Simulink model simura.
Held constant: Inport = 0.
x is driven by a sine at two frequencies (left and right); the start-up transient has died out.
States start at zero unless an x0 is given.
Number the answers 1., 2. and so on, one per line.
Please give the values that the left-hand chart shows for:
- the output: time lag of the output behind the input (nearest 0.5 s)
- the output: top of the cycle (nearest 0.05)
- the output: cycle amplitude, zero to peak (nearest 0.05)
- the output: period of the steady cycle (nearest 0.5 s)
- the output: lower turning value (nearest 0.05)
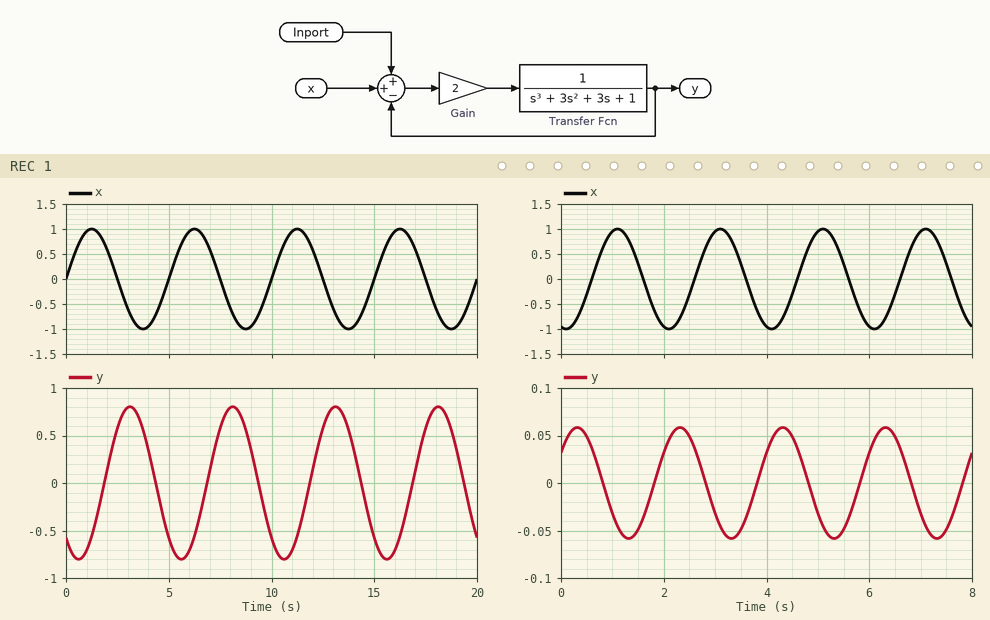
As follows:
1. 2.0 s
2. 0.80
3. 0.80
4. 5.0 s
5. -0.80
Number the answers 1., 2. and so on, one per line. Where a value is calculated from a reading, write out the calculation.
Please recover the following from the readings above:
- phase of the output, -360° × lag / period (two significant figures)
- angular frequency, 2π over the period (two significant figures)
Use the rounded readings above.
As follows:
1. -360 × 2 / 5 = -140°
2. 2π / 5 = 1.3 rad/s
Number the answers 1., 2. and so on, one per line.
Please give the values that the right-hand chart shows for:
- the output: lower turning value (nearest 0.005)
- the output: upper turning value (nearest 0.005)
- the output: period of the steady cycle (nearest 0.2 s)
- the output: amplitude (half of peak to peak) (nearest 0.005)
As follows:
1. -0.060
2. 0.060
3. 2.0 s
4. 0.060
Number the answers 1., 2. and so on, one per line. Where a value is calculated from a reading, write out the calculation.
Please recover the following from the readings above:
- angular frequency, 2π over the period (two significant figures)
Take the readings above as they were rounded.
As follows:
1. 2π / 2 = 3.1 rad/s
